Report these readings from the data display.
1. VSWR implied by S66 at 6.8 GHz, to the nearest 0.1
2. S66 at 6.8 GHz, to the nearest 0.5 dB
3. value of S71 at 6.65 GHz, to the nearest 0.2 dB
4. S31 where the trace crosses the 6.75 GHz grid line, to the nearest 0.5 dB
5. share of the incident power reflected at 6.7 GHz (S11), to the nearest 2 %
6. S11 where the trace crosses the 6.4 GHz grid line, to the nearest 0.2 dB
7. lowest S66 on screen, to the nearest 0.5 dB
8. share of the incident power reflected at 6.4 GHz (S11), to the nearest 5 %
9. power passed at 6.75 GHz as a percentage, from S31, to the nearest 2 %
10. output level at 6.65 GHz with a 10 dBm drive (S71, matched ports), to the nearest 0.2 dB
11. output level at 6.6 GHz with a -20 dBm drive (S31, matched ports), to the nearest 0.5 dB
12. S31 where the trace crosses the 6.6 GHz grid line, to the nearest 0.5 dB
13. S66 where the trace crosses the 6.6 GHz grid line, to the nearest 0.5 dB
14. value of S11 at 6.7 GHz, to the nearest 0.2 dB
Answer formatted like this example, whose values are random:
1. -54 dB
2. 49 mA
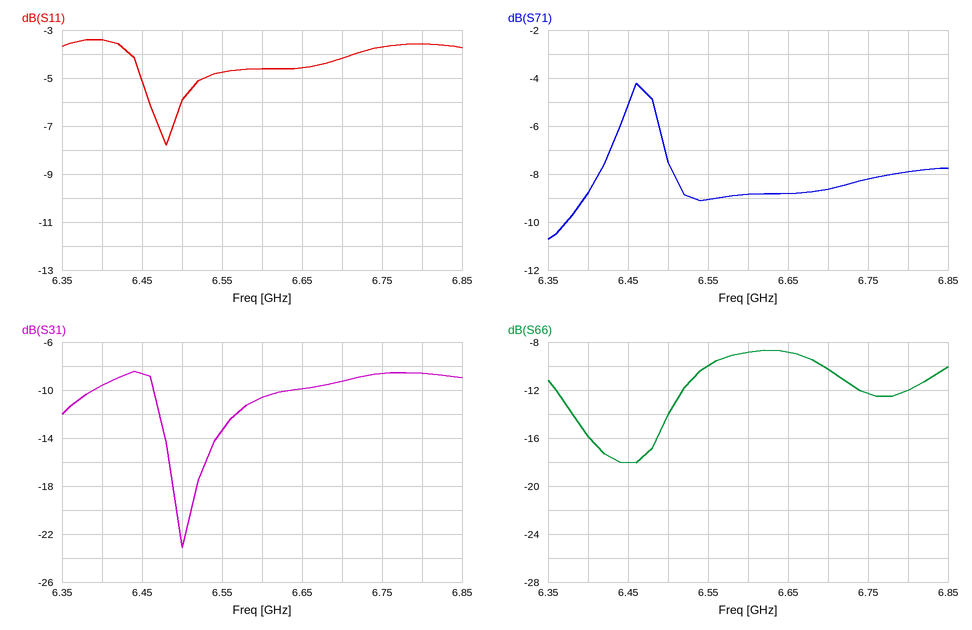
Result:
1. 1.7
2. -12.0 dB
3. -8.8 dB
4. -8.5 dB
5. 38 %
6. -3.4 dB
7. -18.0 dB
8. 45 %
9. 14 %
10. 1.2 dBm
11. -30.5 dBm
12. -10.5 dB
13. -9.0 dB
14. -4.2 dB
